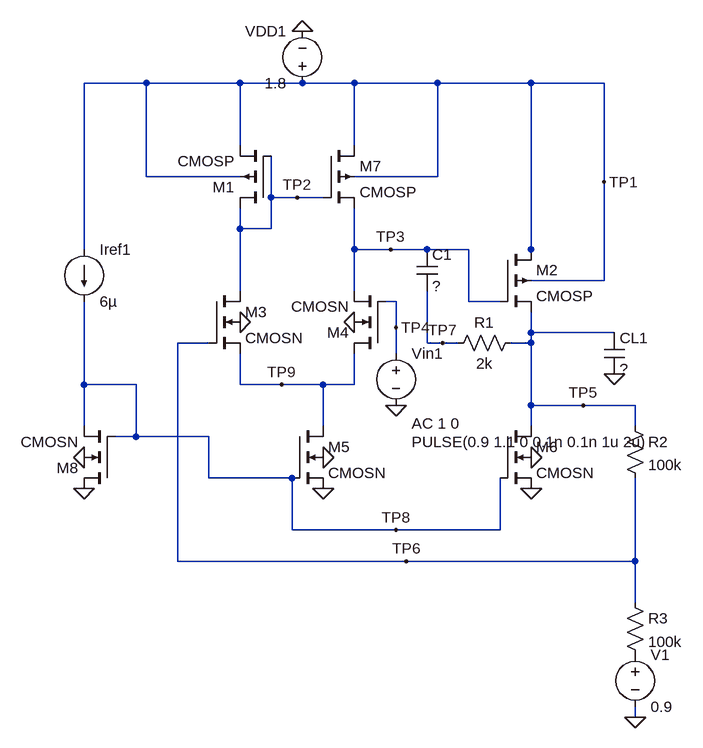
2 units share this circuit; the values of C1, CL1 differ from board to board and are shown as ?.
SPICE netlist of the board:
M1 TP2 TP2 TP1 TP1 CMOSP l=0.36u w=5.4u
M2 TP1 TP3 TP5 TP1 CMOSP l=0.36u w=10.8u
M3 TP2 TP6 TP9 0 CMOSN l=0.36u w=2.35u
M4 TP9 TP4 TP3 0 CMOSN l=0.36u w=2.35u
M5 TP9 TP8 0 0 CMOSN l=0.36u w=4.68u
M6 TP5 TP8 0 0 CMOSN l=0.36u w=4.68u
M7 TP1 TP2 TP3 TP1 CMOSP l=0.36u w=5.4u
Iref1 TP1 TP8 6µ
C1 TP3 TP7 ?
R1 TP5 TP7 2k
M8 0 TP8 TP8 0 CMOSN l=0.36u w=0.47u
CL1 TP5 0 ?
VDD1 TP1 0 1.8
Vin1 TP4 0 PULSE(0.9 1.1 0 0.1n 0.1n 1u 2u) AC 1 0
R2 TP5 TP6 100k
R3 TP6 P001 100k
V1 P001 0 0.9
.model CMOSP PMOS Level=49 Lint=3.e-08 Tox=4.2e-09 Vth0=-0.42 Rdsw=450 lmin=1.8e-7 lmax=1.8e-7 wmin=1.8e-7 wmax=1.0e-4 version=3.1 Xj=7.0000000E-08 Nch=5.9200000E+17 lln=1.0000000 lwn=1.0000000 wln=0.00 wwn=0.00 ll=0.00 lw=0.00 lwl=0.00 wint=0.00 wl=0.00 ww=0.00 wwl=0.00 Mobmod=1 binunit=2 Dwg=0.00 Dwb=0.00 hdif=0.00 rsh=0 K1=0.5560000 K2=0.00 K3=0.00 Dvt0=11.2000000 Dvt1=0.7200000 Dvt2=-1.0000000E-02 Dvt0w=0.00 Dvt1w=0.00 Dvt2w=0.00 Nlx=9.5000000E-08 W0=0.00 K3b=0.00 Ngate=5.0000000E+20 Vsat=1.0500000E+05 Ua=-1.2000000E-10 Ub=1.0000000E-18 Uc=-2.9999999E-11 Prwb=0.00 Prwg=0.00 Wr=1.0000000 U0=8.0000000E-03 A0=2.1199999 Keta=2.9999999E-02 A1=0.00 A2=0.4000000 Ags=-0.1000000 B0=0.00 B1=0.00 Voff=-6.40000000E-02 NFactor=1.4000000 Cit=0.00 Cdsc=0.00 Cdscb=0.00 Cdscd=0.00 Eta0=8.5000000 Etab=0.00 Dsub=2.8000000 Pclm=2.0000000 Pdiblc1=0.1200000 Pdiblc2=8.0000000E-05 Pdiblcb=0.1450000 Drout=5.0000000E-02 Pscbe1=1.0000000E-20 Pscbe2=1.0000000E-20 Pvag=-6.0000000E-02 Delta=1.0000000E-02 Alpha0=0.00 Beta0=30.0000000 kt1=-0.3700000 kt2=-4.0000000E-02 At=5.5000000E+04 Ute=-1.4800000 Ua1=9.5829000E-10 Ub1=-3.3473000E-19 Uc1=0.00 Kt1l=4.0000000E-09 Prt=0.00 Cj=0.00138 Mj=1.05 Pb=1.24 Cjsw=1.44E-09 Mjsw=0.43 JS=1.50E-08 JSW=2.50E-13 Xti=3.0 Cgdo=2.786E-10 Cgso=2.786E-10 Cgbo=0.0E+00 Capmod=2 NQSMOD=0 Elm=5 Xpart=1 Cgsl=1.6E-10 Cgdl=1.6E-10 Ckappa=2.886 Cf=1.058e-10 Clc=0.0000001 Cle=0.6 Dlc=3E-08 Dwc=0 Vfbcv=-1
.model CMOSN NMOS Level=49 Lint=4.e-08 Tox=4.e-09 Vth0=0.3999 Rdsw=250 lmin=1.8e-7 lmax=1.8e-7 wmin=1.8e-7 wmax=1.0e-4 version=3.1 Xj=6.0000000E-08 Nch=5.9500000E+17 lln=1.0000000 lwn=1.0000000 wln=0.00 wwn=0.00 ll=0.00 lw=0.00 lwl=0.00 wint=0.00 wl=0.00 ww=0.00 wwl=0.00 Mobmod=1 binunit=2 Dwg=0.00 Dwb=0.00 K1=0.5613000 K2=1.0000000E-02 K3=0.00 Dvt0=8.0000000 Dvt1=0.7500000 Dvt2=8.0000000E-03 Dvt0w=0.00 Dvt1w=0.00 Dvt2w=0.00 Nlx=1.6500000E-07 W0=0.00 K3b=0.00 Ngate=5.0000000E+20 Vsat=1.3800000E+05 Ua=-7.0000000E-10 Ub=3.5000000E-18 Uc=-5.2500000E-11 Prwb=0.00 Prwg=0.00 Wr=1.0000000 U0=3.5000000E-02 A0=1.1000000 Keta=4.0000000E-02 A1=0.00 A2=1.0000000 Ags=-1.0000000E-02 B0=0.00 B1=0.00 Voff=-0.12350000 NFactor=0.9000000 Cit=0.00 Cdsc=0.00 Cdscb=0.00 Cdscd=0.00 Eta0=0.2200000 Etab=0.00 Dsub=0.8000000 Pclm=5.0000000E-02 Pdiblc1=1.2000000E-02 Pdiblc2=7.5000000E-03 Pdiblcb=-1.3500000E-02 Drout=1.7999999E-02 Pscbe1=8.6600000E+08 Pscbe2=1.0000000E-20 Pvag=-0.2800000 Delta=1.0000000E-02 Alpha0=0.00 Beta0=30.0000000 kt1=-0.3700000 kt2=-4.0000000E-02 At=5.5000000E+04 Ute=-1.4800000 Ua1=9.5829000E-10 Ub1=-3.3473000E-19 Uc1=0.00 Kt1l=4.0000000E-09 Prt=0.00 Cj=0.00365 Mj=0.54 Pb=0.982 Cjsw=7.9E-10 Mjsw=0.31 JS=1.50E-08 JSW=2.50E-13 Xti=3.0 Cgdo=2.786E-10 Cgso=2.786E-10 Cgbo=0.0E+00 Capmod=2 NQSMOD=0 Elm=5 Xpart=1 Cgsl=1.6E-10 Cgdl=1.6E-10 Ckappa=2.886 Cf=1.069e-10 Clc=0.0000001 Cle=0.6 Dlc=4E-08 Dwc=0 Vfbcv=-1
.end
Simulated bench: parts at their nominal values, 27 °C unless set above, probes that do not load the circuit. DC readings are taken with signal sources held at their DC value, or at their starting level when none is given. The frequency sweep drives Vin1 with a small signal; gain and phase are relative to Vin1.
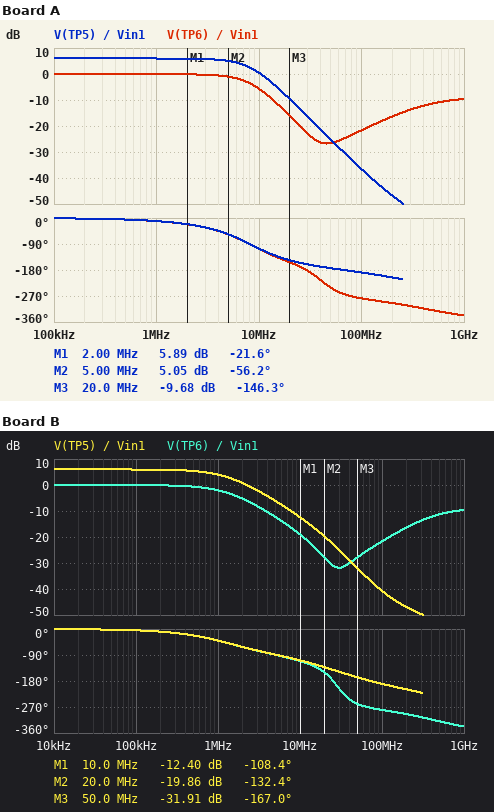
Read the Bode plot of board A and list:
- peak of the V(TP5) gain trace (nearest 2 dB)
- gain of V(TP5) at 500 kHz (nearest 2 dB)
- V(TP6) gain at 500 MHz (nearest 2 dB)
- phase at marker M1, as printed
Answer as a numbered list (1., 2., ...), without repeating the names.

1. 6 dB
2. 6 dB
3. -12 dB
4. -21.6 deg
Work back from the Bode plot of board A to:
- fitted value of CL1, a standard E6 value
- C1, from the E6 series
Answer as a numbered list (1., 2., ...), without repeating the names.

1. 6.8 pF
2. 3.3 pF
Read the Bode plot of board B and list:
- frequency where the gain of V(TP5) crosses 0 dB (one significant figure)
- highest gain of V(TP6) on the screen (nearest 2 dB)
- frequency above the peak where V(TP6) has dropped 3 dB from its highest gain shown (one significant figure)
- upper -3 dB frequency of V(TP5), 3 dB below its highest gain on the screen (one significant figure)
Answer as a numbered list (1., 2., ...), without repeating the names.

1. 2 MHz
2. 0 dB
3. 1 MHz
4. 1 MHz
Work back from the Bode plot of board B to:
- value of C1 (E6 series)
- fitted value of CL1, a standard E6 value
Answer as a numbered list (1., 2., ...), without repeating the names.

1. 15 pF
2. 3.3 pF
